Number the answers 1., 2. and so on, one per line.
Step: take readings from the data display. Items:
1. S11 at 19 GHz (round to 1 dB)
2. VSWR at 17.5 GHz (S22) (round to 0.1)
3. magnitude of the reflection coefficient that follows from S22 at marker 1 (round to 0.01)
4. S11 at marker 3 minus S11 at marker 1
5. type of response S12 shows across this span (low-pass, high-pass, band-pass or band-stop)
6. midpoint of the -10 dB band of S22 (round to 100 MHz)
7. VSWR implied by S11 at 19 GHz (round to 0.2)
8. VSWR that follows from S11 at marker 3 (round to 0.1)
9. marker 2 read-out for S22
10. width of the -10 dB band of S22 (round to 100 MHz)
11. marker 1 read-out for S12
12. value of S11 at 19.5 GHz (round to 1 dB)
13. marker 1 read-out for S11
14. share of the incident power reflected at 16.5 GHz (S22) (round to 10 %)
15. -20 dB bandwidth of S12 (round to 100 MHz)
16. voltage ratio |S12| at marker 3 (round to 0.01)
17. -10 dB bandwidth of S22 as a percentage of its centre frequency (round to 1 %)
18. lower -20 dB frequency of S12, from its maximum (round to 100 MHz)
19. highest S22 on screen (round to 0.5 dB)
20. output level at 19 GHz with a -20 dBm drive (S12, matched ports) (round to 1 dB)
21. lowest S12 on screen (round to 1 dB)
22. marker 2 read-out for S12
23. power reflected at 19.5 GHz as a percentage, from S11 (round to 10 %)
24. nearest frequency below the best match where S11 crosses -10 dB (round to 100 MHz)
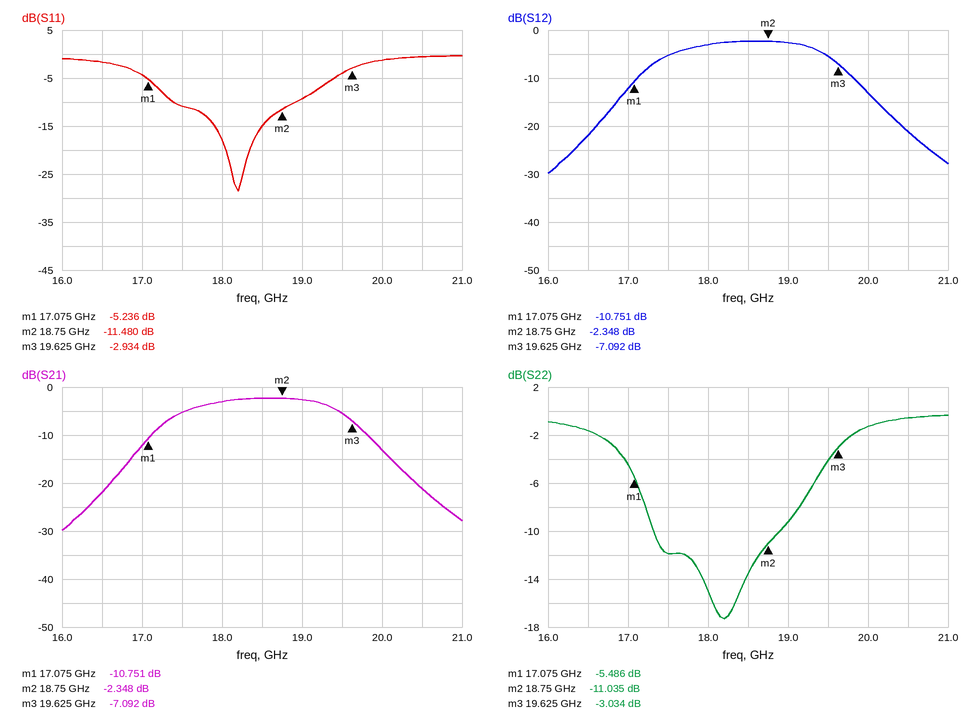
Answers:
1. -9 dB
2. 1.7
3. 0.53
4. 2.302 dB
5. band-pass
6. 18.1 GHz
7. 2.0
8. 6.0
9. -11.035 dB
10. 1.6 GHz
11. -10.751 dB
12. -4 dB
13. -5.236 dB
14. 70 %
15. 4.1 GHz
16. 0.44
17. 9 %
18. 16.5 GHz
19. -0.5 dB
20. -23 dBm
21. -30 dB
22. -2.348 dB
23. 40 %
24. 17.4 GHz
